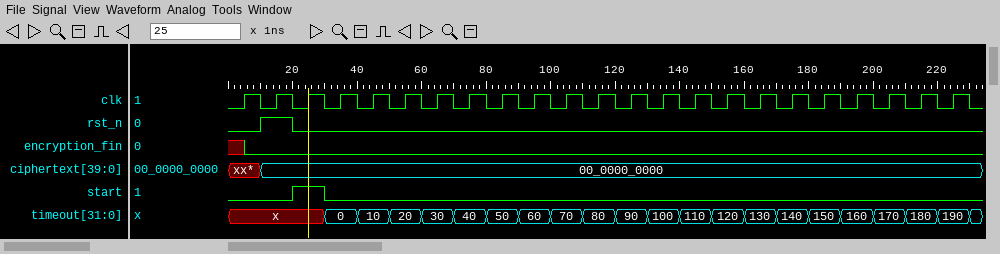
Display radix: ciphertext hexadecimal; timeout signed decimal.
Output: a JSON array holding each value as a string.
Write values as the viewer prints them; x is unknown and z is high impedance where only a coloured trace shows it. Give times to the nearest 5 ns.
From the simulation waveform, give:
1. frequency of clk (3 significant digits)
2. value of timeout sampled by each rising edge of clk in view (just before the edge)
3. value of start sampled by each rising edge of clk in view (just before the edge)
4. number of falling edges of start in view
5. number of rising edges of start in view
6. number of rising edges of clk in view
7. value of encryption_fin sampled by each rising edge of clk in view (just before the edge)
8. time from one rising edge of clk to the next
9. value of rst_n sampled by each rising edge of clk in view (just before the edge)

["100 MHz", "x, x, x, 0, 10, 20, 30, 40, 50, 60, 70, 80, 90, 100, 110, 120, 130, 140, 150, 160, 170, 180, 190", "0 0 1 0 0 0 0 0 0 0 0 0 0 0 0 0 0 0 0 0 0 0 0", "1", "1", "23", "x 0 0 0 0 0 0 0 0 0 0 0 0 0 0 0 0 0 0 0 0 0 0", "10 ns", "0 1 0 0 0 0 0 0 0 0 0 0 0 0 0 0 0 0 0 0 0 0 0"]
